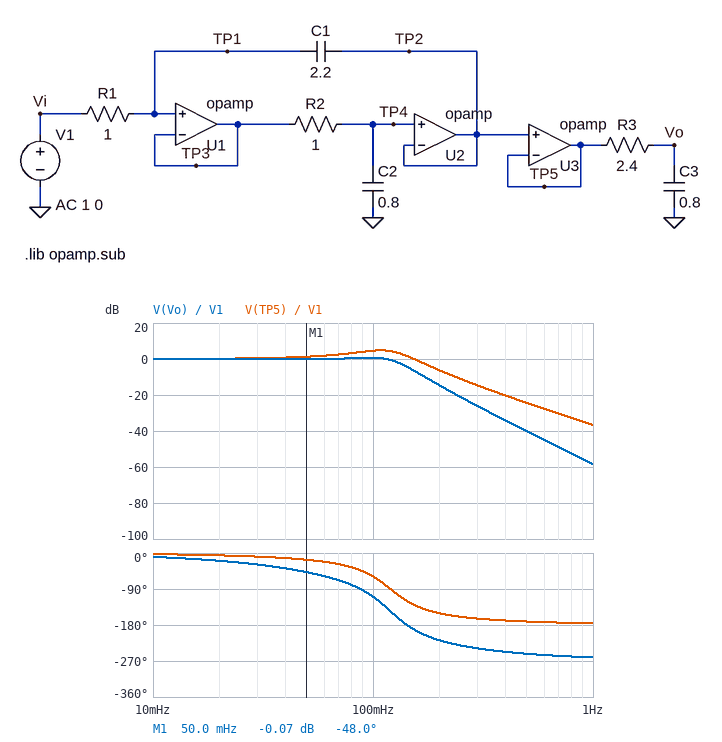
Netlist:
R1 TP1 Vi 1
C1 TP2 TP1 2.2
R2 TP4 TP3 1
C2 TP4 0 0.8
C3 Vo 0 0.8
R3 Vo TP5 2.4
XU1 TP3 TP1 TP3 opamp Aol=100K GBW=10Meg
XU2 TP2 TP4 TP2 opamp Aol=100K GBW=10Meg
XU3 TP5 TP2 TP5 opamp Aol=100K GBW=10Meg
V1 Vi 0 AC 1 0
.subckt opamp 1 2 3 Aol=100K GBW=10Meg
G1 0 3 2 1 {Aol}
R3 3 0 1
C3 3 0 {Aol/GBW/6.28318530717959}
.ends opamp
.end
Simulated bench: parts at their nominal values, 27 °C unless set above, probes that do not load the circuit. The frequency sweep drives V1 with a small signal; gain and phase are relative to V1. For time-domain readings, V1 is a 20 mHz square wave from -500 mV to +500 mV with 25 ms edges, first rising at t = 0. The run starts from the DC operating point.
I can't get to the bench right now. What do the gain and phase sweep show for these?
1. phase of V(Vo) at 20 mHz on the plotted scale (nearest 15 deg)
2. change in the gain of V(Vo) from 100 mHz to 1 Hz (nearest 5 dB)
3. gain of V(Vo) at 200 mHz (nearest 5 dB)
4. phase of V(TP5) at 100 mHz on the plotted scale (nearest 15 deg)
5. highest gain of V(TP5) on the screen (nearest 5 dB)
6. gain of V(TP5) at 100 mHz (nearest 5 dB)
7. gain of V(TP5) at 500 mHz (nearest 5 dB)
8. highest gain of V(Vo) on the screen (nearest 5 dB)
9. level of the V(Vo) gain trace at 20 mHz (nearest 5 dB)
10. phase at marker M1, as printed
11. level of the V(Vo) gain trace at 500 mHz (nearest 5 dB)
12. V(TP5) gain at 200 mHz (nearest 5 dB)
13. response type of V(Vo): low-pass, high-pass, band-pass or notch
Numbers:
-15 deg
-60 dB
-15 dB
-60 deg
5 dB
5 dB
-25 dB
0 dB
0 dB
-48.0 deg
-40 dB
-5 dB
low-pass
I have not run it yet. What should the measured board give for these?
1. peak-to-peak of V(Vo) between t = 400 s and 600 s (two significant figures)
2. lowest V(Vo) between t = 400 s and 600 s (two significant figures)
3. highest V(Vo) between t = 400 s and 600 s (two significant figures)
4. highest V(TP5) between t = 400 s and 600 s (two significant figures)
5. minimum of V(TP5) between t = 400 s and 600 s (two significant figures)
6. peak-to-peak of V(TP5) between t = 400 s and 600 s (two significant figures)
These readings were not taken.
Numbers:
1.3 V
-630 mV
630 mV
870 mV
-870 mV
1.7 V
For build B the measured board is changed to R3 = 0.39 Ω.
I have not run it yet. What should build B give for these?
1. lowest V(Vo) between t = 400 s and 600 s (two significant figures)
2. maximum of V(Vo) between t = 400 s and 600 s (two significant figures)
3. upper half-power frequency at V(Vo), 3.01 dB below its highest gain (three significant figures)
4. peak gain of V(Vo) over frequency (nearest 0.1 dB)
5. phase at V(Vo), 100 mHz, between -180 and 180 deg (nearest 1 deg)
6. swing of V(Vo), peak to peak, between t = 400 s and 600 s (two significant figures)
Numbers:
-860 mV
860 mV
141 mHz
4.6 dB
-70 deg
1.7 V
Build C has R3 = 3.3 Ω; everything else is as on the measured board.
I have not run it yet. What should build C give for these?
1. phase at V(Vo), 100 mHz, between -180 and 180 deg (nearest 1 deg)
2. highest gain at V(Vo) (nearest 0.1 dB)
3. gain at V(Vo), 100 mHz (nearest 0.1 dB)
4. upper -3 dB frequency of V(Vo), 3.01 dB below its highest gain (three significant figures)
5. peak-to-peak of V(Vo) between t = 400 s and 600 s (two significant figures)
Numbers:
-118 deg
0 dB
-1.1 dB
123 mHz
1.1 V
